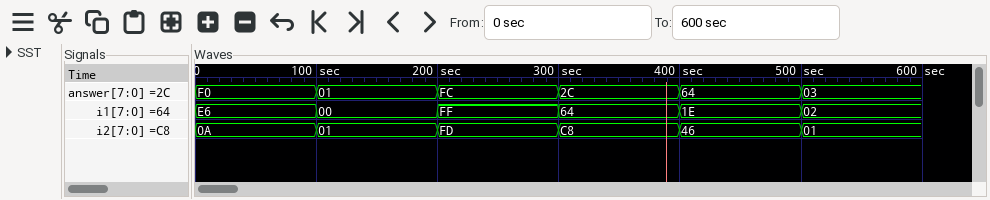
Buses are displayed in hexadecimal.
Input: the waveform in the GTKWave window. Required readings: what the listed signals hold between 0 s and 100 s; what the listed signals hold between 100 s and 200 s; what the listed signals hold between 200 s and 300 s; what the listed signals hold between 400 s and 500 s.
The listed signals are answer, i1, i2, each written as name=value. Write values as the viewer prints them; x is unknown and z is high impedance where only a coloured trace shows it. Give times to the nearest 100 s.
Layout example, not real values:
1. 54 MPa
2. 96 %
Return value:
1. answer=F0, i1=E6, i2=0A
2. answer=01, i1=00, i2=01
3. answer=FC, i1=FF, i2=FD
4. answer=64, i1=1E, i2=46
